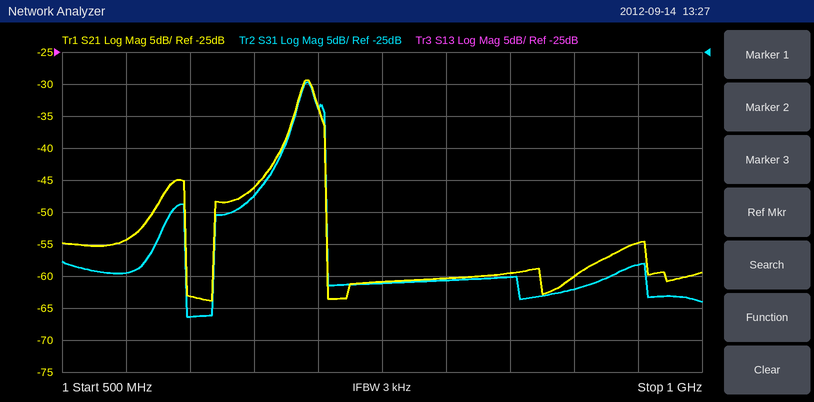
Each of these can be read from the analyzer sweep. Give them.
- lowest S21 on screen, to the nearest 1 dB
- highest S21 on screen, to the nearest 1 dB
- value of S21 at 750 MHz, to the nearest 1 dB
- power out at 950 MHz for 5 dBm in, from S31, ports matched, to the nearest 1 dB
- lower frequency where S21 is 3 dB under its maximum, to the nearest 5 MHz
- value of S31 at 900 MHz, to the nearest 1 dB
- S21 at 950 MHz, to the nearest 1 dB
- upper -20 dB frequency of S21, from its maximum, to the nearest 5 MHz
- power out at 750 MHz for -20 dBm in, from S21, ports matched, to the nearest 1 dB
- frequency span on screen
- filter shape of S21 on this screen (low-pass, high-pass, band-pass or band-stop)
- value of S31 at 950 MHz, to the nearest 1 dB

-64 dB
-29 dB
-61 dB
-53 dBm
685 MHz
-62 dB
-55 dB
705 MHz
-81 dBm
500 MHz
band-pass
-58 dB
